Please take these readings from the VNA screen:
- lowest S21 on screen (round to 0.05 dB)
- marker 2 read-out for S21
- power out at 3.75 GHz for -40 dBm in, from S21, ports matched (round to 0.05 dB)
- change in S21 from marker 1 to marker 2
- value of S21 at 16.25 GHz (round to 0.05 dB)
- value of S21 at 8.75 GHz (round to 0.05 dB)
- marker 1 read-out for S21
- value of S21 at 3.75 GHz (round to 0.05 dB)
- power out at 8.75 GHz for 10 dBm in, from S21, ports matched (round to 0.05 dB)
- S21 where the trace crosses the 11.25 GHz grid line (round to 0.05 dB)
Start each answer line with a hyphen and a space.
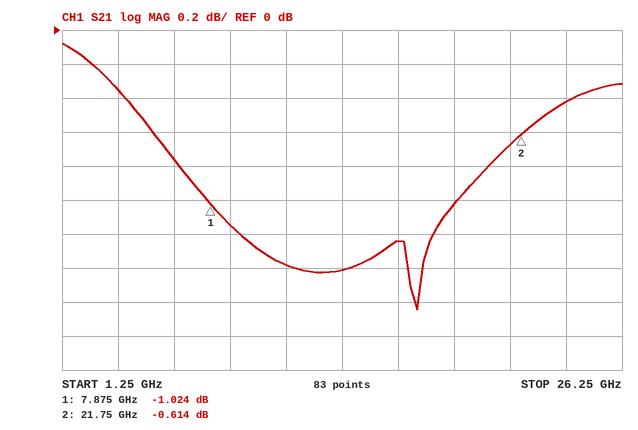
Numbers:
- -1.65 dB
- -0.614 dB
- -40.35 dBm
- 0.410 dB
- -1.25 dB
- -1.15 dB
- -1.024 dB
- -0.35 dB
- 8.85 dBm
- -1.40 dB
